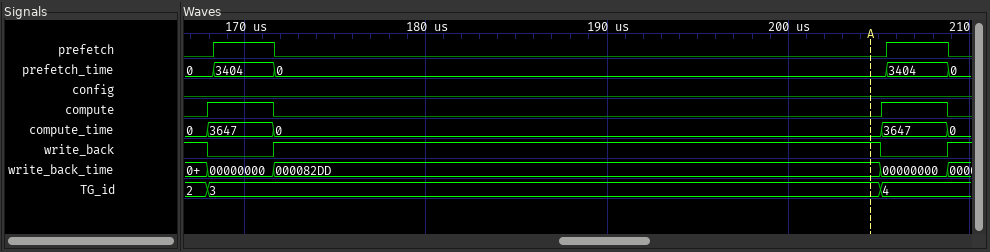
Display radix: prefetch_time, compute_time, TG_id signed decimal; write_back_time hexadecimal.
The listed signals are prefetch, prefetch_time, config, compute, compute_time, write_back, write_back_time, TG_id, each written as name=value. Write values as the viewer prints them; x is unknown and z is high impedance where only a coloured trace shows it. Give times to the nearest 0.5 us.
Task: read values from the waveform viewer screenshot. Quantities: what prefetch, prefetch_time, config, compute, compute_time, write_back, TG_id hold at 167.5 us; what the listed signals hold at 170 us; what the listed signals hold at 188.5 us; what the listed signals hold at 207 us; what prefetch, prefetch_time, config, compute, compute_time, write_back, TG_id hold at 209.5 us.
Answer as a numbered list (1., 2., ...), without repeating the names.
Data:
1. prefetch=0, prefetch_time=0, config=0, compute=0, compute_time=0, write_back=1, TG_id=2
2. prefetch=1, prefetch_time=3404, config=0, compute=1, compute_time=3647, write_back=0, write_back_time=00000000, TG_id=3
3. prefetch=0, prefetch_time=0, config=0, compute=0, compute_time=0, write_back=1, write_back_time=000082DD, TG_id=3
4. prefetch=1, prefetch_time=3404, config=0, compute=1, compute_time=3647, write_back=0, write_back_time=00000000, TG_id=4
5. prefetch=0, prefetch_time=0, config=0, compute=0, compute_time=0, write_back=1, TG_id=4
